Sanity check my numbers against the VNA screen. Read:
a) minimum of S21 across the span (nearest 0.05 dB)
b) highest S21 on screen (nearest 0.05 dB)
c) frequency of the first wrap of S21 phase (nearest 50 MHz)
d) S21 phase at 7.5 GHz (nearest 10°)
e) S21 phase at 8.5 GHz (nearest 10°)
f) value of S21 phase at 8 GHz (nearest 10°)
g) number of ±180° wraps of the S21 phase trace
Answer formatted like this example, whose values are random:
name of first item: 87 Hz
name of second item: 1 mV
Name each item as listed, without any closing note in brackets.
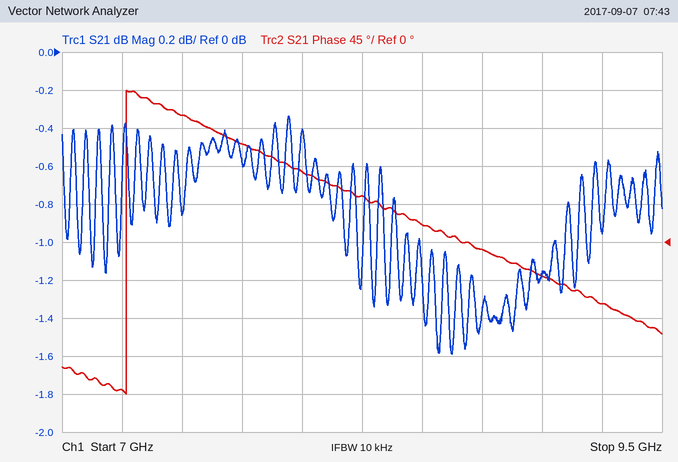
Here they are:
minimum of S21 across the span: -1.60 dB
highest S21 on screen: -0.35 dB
frequency of the first wrap of S21 phase: 7.25 GHz
S21 phase at 7.5 GHz: 150°
S21 phase at 8.5 GHz: 20°
value of S21 phase at 8 GHz: 80°
number of ±180° wraps of the S21 phase trace: 1
